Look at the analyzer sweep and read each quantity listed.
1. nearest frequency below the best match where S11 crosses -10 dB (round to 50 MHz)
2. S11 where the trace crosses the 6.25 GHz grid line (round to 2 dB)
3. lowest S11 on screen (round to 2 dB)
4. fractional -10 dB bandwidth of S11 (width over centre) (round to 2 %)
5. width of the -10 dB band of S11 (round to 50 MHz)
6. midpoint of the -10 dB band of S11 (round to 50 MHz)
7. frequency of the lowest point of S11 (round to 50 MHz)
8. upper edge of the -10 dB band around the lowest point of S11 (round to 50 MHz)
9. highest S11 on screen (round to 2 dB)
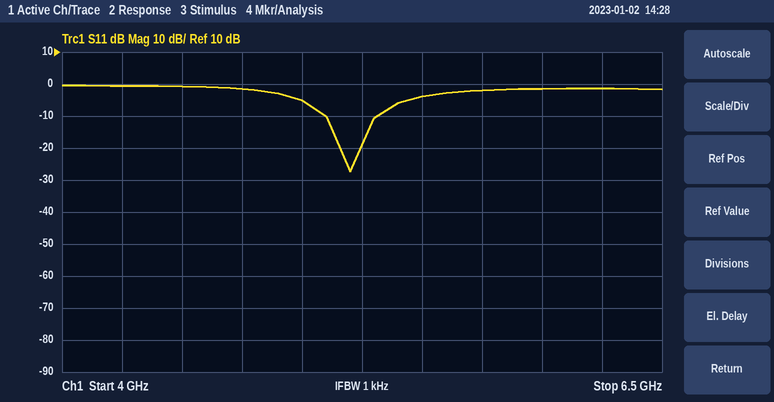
5.10 GHz
-2 dB
-28 dB
4 %
200 MHz
5.20 GHz
5.20 GHz
5.30 GHz
0 dB
